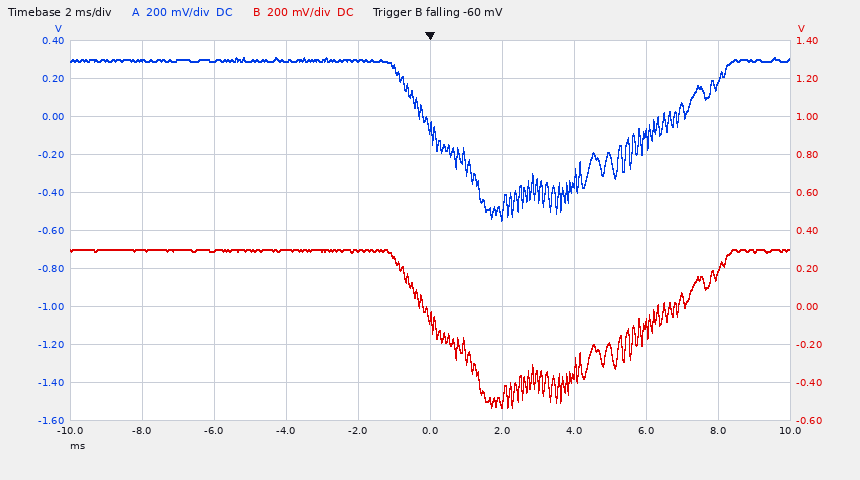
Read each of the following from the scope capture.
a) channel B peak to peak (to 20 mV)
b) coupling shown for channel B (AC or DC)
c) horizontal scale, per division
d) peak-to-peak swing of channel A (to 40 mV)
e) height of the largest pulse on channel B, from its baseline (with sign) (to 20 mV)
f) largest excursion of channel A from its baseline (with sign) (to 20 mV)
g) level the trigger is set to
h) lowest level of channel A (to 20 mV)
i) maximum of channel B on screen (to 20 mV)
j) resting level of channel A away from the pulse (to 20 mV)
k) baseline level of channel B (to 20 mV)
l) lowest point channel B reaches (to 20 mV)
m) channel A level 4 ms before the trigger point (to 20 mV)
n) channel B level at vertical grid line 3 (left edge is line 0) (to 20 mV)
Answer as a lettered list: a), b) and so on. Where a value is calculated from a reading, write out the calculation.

a) 300 mV − (-540 mV) = 840 mV
b) DC
c) 2 ms
d) 840 mV
e) -540 mV − (300 mV) = -840 mV
f) -540 mV − (300 mV) = -840 mV
g) -60 mV
h) -540 mV
i) 300 mV
j) 300 mV
k) 300 mV
l) -540 mV
m) 300 mV
n) 300 mV
